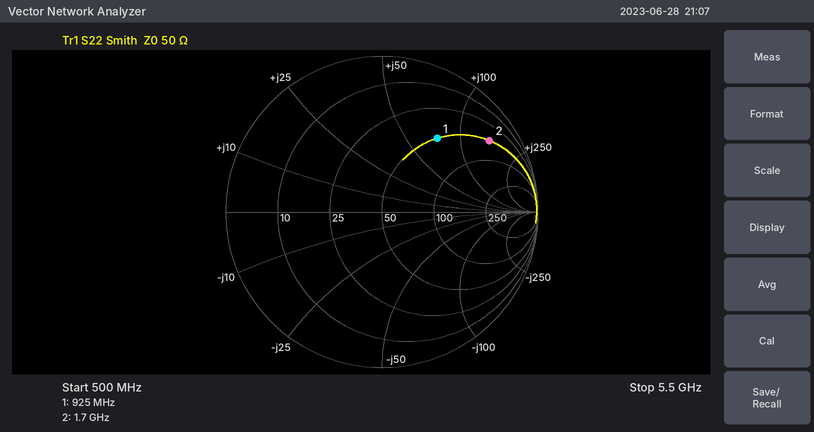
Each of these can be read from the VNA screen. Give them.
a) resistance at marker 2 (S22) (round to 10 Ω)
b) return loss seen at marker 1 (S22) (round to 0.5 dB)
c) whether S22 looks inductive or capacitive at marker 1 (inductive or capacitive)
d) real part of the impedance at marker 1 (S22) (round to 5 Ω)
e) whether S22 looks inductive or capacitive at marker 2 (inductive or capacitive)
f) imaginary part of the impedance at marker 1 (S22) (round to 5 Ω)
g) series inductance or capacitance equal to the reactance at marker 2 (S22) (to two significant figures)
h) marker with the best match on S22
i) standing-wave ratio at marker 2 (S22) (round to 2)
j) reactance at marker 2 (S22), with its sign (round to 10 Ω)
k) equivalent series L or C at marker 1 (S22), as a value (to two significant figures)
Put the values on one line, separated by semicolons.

50 Ω; 4.5 dB; inductive; 50 Ω; inductive; +75 Ω; 14 nH; marker 1; 10; +150 Ω; 13 nH
